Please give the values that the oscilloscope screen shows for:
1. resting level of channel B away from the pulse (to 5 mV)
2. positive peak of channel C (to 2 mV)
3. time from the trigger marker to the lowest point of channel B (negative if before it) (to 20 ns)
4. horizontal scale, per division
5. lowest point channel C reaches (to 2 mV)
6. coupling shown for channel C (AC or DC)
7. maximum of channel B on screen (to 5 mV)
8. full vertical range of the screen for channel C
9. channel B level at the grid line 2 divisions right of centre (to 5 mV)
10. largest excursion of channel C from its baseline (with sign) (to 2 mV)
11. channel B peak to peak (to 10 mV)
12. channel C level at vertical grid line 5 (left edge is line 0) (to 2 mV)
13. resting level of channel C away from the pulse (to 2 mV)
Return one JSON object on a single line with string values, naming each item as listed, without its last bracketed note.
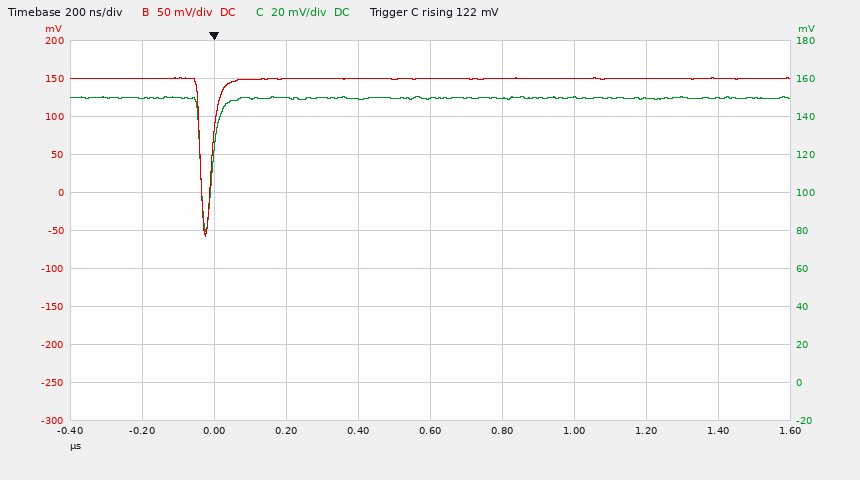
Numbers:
{"resting level of channel B away from the pulse": "150 mV", "positive peak of channel C": "150 mV", "time from the trigger marker to the lowest point of channel B (negative if before it)": "-20 ns", "horizontal scale, per division": "200 ns", "lowest point channel C reaches": "80 mV", "coupling shown for channel C": "DC", "maximum of channel B on screen": "150 mV", "full vertical range of the screen for channel C": "200 mV", "channel B level at the grid line 2 divisions right of centre": "150 mV", "largest excursion of channel C from its baseline (with sign)": "-70 mV", "channel B peak to peak": "210 mV", "channel C level at vertical grid line 5 (left edge is line 0)": "150 mV", "resting level of channel C away from the pulse": "150 mV"}
